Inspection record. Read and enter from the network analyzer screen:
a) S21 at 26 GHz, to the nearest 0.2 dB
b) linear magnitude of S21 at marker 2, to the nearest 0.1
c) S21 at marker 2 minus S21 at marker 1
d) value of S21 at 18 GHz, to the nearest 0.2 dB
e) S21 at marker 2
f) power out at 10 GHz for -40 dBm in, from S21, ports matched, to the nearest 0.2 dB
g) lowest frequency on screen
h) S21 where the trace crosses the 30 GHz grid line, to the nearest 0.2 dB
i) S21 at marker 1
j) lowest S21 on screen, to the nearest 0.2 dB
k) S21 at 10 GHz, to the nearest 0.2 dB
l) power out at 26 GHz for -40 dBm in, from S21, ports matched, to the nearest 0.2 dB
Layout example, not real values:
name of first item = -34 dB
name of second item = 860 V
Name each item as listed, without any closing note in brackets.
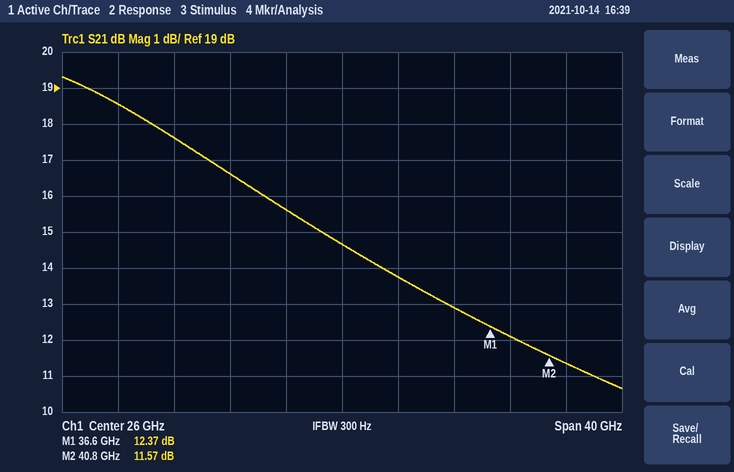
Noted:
S21 at 26 GHz, to the nearest 0.2 dB = 14.6 dB
linear magnitude of S21 at marker 2, to the nearest 0.1 = 3.8
S21 at marker 2 minus S21 at marker 1 = -0.80 dB
value of S21 at 18 GHz, to the nearest 0.2 dB = 16.6 dB
S21 at marker 2 = 11.57 dB
power out at 10 GHz for -40 dBm in, from S21, ports matched, to the nearest 0.2 dB = -21.4 dBm
lowest frequency on screen = 6 GHz
S21 where the trace crosses the 30 GHz grid line, to the nearest 0.2 dB = 13.8 dB
S21 at marker 1 = 12.37 dB
lowest S21 on screen, to the nearest 0.2 dB = 10.6 dB
S21 at 10 GHz, to the nearest 0.2 dB = 18.6 dB
power out at 26 GHz for -40 dBm in, from S21, ports matched, to the nearest 0.2 dB = -25.4 dBm
